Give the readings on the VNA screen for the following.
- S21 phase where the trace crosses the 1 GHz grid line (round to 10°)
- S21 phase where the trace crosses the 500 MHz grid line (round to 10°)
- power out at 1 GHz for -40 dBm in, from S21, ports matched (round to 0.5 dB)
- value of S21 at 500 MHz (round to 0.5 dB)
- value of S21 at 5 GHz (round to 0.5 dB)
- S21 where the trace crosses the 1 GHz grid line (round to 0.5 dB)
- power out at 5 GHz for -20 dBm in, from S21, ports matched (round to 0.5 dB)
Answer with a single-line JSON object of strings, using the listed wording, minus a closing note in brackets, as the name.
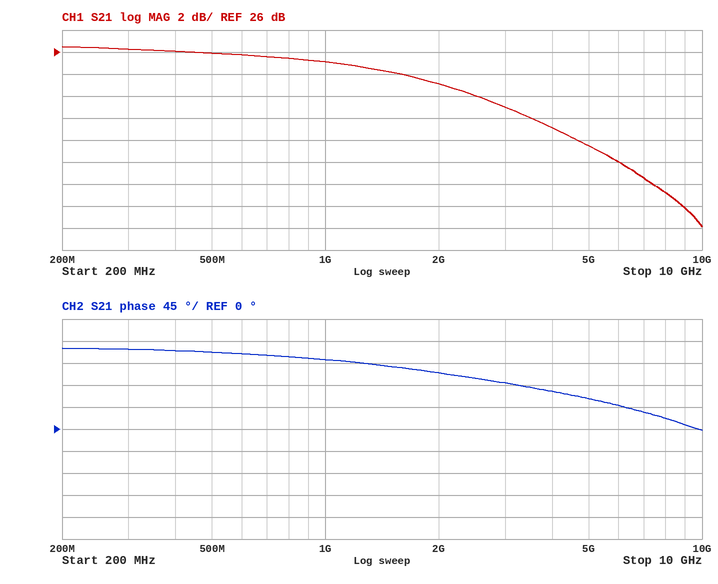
{"S21 phase where the trace crosses the 1 GHz grid line": "140°", "S21 phase where the trace crosses the 500 MHz grid line": "160°", "power out at 1 GHz for -40 dBm in, from S21, ports matched": "-15.0 dBm", "value of S21 at 500 MHz": "26.0 dB", "value of S21 at 5 GHz": "17.5 dB", "S21 where the trace crosses the 1 GHz grid line": "25.0 dB", "power out at 5 GHz for -20 dBm in, from S21, ports matched": "-2.5 dBm"}
